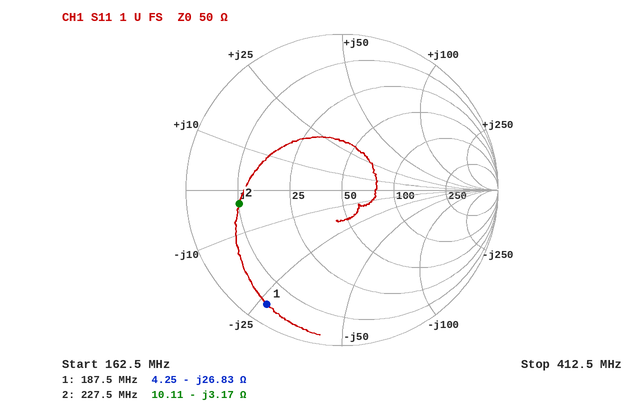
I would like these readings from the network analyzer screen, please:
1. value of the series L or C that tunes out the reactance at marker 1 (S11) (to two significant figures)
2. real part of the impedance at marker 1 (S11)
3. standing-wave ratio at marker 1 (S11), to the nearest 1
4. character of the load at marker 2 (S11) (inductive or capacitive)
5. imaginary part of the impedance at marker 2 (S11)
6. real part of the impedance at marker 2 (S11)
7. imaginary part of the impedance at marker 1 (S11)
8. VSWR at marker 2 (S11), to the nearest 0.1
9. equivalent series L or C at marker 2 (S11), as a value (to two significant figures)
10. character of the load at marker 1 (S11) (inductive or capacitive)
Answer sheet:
23 nH
4.25 Ω
15
capacitive
-3.17 Ω
10.11 Ω
-26.83 Ω
5.0
220 pF
capacitive
